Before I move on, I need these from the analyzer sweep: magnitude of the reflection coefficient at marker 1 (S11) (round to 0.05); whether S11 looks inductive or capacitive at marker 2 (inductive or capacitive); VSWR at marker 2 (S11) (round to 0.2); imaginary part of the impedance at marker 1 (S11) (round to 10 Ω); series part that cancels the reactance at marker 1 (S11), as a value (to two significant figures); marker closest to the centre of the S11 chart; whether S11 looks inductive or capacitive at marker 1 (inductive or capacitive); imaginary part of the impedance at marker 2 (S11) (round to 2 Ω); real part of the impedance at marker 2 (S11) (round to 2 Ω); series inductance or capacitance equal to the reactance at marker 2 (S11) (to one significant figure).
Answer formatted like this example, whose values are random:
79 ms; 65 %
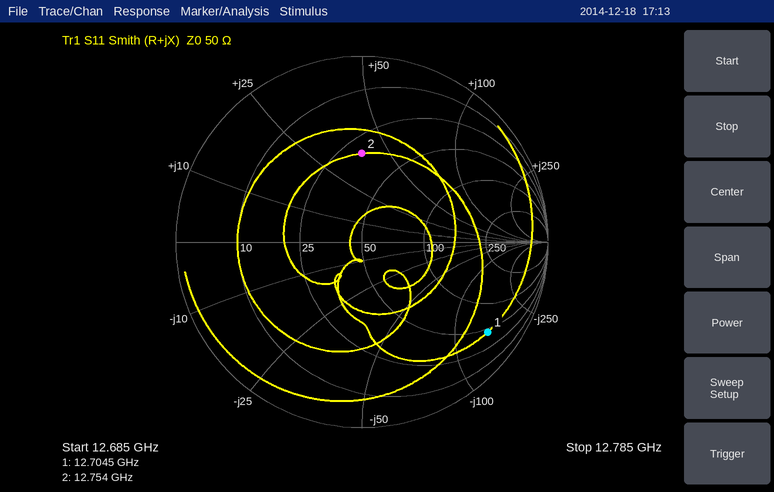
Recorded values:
0.85; inductive; 2.8; -140 Ω; 1.8 nH; marker 2; capacitive; +38 Ω; 32 Ω; 500 pH
